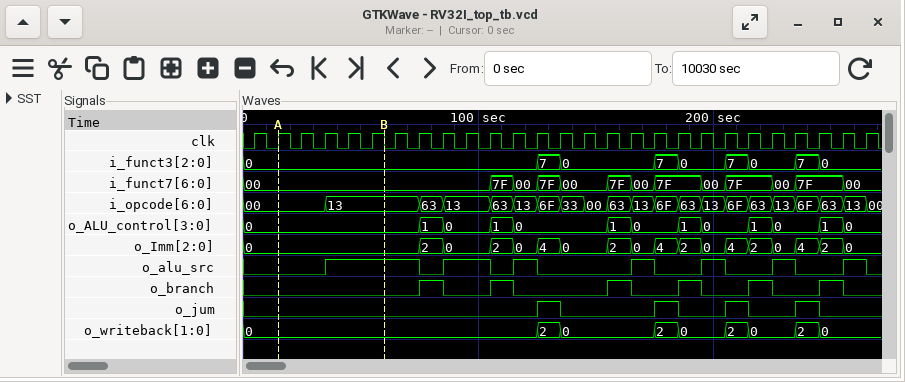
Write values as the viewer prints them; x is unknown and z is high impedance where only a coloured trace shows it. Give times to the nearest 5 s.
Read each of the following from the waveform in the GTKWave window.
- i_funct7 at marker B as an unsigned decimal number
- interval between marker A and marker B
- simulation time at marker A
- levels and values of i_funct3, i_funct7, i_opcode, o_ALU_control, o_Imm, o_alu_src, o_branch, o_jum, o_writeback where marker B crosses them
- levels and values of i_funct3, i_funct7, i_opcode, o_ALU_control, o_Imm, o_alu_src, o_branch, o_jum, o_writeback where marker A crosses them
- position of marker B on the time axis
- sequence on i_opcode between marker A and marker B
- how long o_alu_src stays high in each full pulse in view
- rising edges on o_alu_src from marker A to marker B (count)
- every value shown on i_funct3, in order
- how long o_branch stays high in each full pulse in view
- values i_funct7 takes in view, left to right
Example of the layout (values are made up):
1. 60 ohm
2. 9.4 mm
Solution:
1. 0
2. 45 s
3. 15 s
4. i_funct3=0, i_funct7=00, i_opcode=13, o_ALU_control=0, o_Imm=0, o_alu_src=1, o_branch=0, o_jum=0, o_writeback=0
5. i_funct3=0, i_funct7=00, i_opcode=00, o_ALU_control=0, o_Imm=0, o_alu_src=0, o_branch=0, o_jum=0, o_writeback=0
6. 60 s
7. 00, 13
8. 40 s, 20 s, 10 s, 10 s, 10 s, 10 s, 10 s
9. 1
10. 0, 7, 0, 7, 0, 7, 0, 7, 0
11. 10 s, 10 s, 10 s, 10 s, 10 s, 10 s
12. 00, 7F, 00, 7F, 00, 7F, 00, 7F, 00, 7F, 00, 7F, 00
